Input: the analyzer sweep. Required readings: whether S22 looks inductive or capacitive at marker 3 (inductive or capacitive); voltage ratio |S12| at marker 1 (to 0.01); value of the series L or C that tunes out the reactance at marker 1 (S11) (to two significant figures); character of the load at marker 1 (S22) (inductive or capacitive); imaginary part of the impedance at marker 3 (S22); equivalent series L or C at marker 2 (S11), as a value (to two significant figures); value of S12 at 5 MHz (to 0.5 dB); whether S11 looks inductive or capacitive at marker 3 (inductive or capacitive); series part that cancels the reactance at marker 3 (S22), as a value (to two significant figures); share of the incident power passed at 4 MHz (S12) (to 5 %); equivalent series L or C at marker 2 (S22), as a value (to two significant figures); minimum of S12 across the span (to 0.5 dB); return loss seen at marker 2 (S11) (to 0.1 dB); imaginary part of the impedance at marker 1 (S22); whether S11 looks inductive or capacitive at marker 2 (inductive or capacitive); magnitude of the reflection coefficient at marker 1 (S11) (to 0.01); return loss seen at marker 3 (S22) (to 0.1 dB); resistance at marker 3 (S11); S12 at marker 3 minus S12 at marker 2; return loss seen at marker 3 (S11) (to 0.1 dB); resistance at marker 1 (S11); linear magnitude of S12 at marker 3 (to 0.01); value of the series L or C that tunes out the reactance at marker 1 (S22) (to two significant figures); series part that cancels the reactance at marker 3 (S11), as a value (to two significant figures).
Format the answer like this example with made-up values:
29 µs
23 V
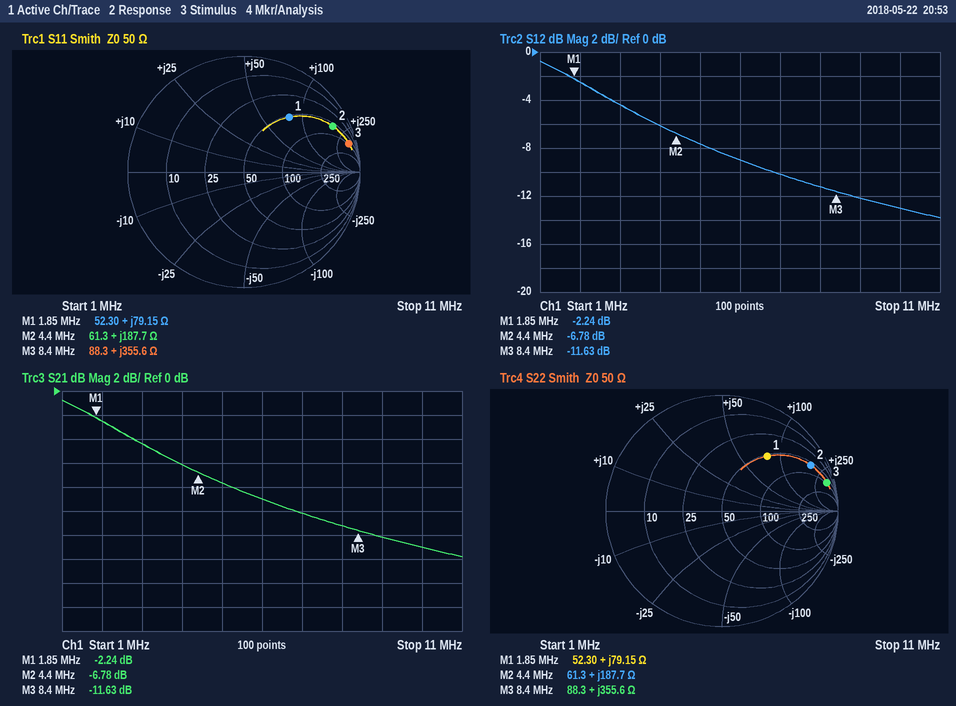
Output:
inductive
0.77
1.1 nF
inductive
+355.6 Ω
6.8 µH
-7.5 dB
inductive
53 pF
25 %
6.8 µH
-14.0 dB
1.3 dB
+79.15 Ω
inductive
0.61
0.6 dB
88.3 Ω
-4.85 dB
0.6 dB
52.30 Ω
0.26
1.1 nF
53 pF
